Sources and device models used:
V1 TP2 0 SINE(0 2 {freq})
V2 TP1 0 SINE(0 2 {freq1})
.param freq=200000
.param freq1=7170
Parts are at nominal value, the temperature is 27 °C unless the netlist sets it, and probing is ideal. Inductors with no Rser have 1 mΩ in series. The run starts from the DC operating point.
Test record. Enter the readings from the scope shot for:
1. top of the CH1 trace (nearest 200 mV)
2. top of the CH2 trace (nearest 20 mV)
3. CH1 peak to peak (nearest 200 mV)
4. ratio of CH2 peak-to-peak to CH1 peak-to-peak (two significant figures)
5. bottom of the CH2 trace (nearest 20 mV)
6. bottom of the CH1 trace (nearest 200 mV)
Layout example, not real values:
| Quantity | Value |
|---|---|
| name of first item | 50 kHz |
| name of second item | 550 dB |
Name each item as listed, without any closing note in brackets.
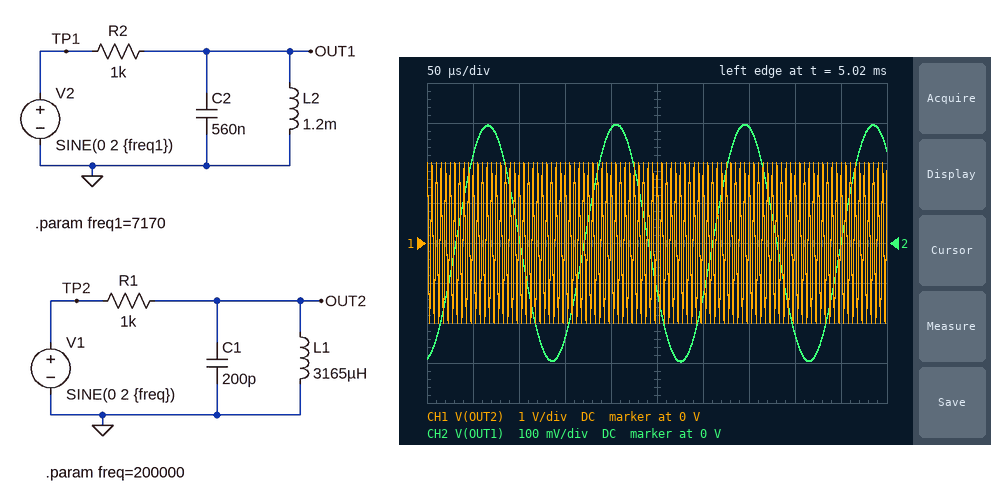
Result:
| Quantity | Value |
|---|---|
| top of the CH1 trace | 2.0 V |
| top of the CH2 trace | 300 mV |
| CH1 peak to peak | 4.0 V |
| ratio of CH2 peak-to-peak to CH1 peak-to-peak | 0.15 |
| bottom of the CH2 trace | -300 mV |
| bottom of the CH1 trace | -2.0 V |
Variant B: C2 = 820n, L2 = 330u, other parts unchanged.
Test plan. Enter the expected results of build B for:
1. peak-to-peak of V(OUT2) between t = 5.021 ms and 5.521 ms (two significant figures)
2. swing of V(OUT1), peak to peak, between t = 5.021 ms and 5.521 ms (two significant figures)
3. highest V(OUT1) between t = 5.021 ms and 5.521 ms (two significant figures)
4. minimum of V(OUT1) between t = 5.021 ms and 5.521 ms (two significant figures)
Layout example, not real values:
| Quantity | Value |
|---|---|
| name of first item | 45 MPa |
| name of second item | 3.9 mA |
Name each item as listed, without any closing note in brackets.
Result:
| Quantity | Value |
|---|---|
| peak-to-peak of V(OUT2) between t = 5.021 ms and 5.521 ms | 4.0 V |
| swing of V(OUT1), peak to peak, between t = 5.021 ms and 5.521 ms | 140 mV |
| highest V(OUT1) between t = 5.021 ms and 5.521 ms | 69 mV |
| minimum of V(OUT1) between t = 5.021 ms and 5.521 ms | -68 mV |
